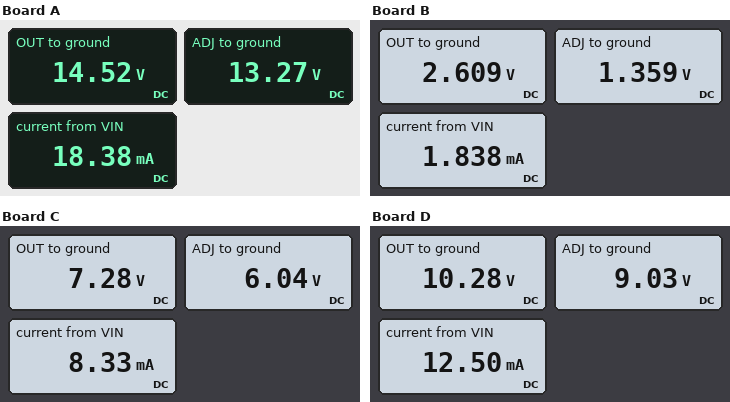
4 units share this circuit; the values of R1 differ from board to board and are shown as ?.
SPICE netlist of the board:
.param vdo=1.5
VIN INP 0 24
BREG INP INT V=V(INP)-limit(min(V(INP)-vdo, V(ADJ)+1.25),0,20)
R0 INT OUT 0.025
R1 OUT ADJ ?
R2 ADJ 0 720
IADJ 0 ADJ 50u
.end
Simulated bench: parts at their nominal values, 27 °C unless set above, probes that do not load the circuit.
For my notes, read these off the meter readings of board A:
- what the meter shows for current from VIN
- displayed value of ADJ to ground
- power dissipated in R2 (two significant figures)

18.38 mA
13.27 V
240 mW
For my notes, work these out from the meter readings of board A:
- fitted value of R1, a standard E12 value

68 Ω
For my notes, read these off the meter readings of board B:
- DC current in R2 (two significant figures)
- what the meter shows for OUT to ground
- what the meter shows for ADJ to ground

1.9 mA
2.609 V
1.359 V
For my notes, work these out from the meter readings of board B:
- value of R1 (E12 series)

680 Ω
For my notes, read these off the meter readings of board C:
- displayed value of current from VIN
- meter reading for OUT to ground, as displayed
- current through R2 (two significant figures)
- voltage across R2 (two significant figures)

8.33 mA
7.28 V
8.4 mA
6.0 V
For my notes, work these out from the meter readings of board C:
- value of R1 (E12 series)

150 Ω
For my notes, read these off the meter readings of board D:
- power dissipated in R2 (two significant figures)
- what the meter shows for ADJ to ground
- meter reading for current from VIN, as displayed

110 mW
9.03 V
12.50 mA
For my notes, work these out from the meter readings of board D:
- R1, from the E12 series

100 Ω
